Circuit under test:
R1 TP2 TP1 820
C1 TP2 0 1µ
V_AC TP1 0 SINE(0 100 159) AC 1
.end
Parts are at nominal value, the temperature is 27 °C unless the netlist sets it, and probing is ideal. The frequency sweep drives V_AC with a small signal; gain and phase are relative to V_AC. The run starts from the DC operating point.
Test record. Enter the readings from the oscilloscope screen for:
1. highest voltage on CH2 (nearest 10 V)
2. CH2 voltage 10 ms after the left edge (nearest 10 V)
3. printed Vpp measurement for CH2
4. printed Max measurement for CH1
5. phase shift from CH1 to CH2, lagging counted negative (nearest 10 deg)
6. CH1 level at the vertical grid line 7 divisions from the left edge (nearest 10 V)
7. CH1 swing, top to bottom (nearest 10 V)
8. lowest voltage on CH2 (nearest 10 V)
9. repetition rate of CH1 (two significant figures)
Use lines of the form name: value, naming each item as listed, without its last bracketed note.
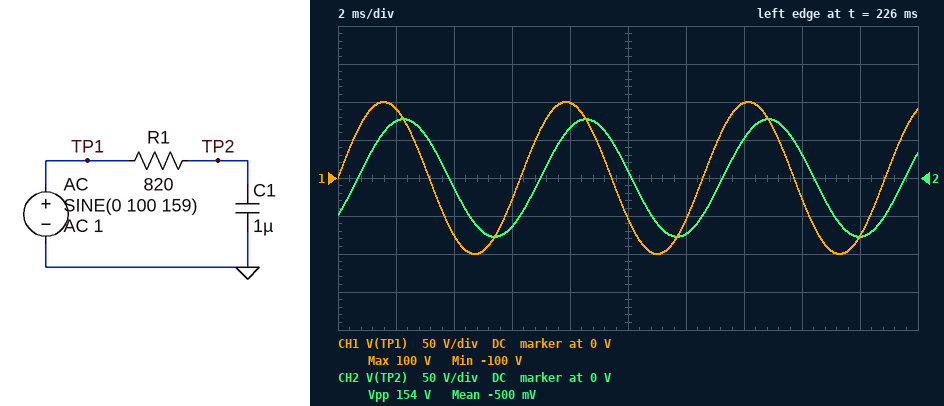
highest voltage on CH2: 80 V
CH2 voltage 10 ms after the left edge: 10 V
printed Vpp measurement for CH2: 154 V
printed Max measurement for CH1: 100 V
phase shift from CH1 to CH2, lagging counted negative: -40 deg
CH1 level at the vertical grid line 7 divisions from the left edge: 100 V
CH1 swing, top to bottom: 200 V
lowest voltage on CH2: -80 V
repetition rate of CH1: 160 Hz
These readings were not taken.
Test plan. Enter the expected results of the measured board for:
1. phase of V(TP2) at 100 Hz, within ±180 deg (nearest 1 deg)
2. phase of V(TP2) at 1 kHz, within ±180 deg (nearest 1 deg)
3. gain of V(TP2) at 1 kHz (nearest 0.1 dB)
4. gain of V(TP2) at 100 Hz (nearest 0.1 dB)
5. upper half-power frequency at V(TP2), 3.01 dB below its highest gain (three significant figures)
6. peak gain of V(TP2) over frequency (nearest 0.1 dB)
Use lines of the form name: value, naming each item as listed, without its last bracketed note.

phase of V(TP2) at 100 Hz, within ±180 deg: -27 deg
phase of V(TP2) at 1 kHz, within ±180 deg: -79 deg
gain of V(TP2) at 1 kHz: -14.4 dB
gain of V(TP2) at 100 Hz: -1.0 dB
upper half-power frequency at V(TP2), 3.01 dB below its highest gain: 194 Hz
peak gain of V(TP2) over frequency: 0 dB
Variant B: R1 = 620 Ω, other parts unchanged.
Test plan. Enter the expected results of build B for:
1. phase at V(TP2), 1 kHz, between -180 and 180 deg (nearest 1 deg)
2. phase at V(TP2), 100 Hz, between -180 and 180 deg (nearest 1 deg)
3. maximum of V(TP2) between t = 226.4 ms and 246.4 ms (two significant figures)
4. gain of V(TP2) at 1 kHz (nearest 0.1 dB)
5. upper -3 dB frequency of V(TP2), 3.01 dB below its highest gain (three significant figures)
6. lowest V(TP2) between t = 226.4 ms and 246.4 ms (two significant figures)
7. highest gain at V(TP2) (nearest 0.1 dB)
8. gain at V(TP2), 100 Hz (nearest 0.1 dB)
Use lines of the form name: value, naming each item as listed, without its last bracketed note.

phase at V(TP2), 1 kHz, between -180 and 180 deg: -76 deg
phase at V(TP2), 100 Hz, between -180 and 180 deg: -21 deg
maximum of V(TP2) between t = 226.4 ms and 246.4 ms: 85 V
gain of V(TP2) at 1 kHz: -12.1 dB
upper -3 dB frequency of V(TP2), 3.01 dB below its highest gain: 257 Hz
lowest V(TP2) between t = 226.4 ms and 246.4 ms: -85 V
highest gain at V(TP2): 0 dB
gain at V(TP2), 100 Hz: -0.6 dB
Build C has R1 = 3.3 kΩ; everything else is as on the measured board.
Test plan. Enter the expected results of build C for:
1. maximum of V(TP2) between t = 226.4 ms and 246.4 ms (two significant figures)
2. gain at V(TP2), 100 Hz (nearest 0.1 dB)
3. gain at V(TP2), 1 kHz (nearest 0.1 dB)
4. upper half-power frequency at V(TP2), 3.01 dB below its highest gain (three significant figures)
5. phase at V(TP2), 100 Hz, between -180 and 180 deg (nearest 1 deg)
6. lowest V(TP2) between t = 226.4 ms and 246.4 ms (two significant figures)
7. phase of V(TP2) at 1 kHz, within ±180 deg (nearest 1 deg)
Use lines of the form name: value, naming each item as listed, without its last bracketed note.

maximum of V(TP2) between t = 226.4 ms and 246.4 ms: 29 V
gain at V(TP2), 100 Hz: -7.2 dB
gain at V(TP2), 1 kHz: -26.3 dB
upper half-power frequency at V(TP2), 3.01 dB below its highest gain: 48.2 Hz
phase at V(TP2), 100 Hz, between -180 and 180 deg: -64 deg
lowest V(TP2) between t = 226.4 ms and 246.4 ms: -29 V
phase of V(TP2) at 1 kHz, within ±180 deg: -87 deg
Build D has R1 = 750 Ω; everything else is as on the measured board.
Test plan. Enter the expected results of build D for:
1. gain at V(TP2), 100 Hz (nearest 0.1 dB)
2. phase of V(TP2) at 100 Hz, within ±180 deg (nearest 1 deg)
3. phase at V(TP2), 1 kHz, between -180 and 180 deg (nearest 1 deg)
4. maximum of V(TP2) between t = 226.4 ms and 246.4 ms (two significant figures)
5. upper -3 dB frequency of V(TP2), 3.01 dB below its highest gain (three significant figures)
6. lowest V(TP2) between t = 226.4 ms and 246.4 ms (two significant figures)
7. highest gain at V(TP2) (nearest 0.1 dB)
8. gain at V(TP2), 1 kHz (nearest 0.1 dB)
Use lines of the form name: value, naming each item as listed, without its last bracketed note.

gain at V(TP2), 100 Hz: -0.9 dB
phase of V(TP2) at 100 Hz, within ±180 deg: -25 deg
phase at V(TP2), 1 kHz, between -180 and 180 deg: -78 deg
maximum of V(TP2) between t = 226.4 ms and 246.4 ms: 80 V
upper -3 dB frequency of V(TP2), 3.01 dB below its highest gain: 212 Hz
lowest V(TP2) between t = 226.4 ms and 246.4 ms: -80 V
highest gain at V(TP2): 0 dB
gain at V(TP2), 1 kHz: -13.7 dB
